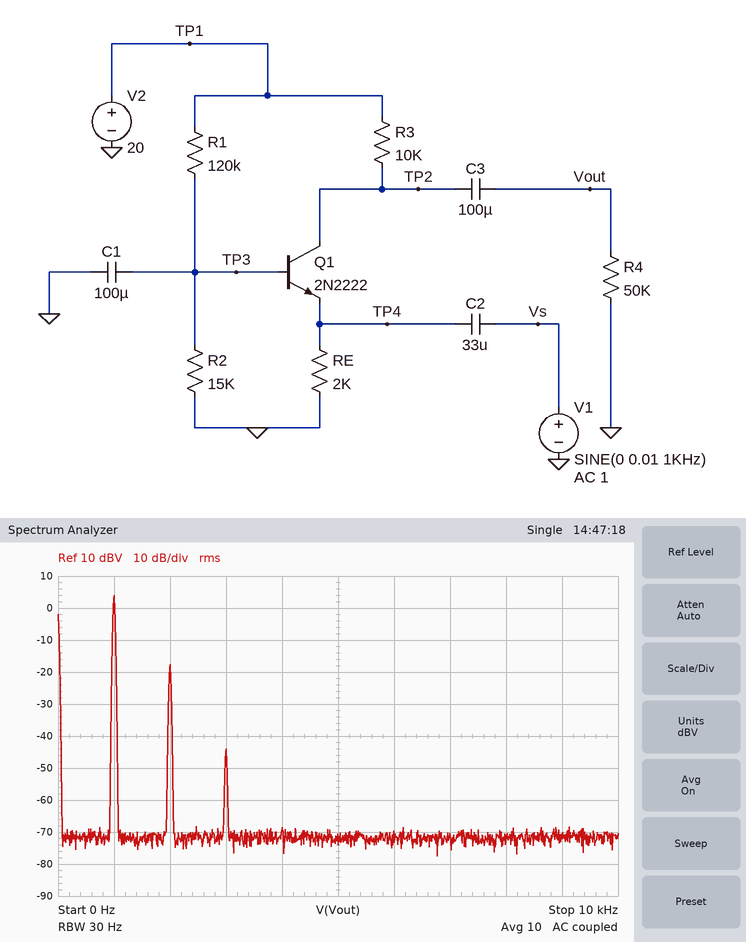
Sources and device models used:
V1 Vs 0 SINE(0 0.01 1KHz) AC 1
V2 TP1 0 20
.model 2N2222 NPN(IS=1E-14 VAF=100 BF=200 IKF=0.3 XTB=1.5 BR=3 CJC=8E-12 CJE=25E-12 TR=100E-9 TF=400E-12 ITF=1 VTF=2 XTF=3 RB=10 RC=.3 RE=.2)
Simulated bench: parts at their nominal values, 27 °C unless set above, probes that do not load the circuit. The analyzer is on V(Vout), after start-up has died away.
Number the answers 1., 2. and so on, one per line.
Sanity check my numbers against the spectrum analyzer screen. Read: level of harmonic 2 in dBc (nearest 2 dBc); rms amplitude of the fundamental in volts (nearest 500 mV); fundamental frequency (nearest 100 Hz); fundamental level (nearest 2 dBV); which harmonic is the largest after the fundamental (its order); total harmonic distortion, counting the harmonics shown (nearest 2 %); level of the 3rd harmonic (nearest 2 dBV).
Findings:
1. -22 dBc
2. 1.5 V
3. 1.0 kHz
4. 4 dBV
5. 2
6. 8 %
7. -44 dBV
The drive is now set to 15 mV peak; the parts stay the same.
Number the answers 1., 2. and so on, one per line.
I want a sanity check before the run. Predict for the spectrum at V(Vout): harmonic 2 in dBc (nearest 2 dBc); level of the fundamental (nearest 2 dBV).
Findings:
1. -18 dBc
2. 8 dBV
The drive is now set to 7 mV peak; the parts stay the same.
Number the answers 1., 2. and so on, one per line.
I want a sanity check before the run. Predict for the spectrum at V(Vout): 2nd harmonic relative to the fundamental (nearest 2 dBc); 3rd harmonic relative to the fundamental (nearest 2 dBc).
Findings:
1. -24 dBc
2. -54 dBc
